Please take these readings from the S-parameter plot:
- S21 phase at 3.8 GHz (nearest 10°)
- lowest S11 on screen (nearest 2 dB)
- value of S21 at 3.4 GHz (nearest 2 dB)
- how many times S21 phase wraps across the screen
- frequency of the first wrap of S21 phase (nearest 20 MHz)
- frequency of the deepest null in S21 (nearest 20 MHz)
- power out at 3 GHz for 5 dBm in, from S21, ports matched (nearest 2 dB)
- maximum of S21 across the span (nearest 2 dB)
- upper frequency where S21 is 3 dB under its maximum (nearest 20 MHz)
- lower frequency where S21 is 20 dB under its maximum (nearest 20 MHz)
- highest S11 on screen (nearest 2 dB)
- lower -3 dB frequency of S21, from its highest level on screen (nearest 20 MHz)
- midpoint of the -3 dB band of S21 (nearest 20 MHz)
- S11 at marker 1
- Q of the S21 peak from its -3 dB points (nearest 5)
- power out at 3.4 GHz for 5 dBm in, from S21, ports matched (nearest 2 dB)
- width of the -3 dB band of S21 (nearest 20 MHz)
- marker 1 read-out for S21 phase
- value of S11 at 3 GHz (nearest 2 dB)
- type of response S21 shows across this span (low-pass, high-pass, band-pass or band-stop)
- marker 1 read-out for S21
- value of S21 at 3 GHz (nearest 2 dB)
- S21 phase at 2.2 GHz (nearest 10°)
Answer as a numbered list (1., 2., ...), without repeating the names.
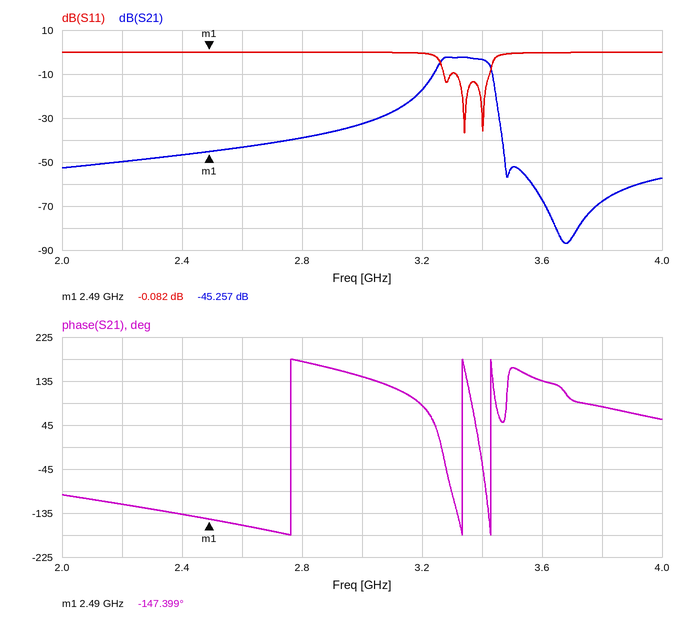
1. 80°
2. -36 dB
3. -4 dB
4. 3
5. 2.76 GHz
6. 3.68 GHz
7. -28 dBm
8. -2 dB
9. 3.42 GHz
10. 3.16 GHz
11. 0 dB
12. 3.26 GHz
13. 3.34 GHz
14. -0.082 dB
15. 20
16. 2 dBm
17. 160 MHz
18. -147.399°
19. 0 dB
20. band-pass
21. -45.257 dB
22. -32 dB
23. -120°
